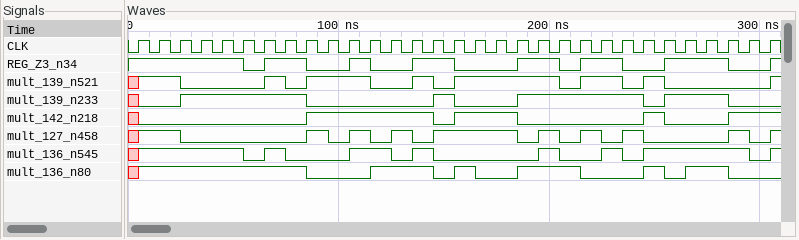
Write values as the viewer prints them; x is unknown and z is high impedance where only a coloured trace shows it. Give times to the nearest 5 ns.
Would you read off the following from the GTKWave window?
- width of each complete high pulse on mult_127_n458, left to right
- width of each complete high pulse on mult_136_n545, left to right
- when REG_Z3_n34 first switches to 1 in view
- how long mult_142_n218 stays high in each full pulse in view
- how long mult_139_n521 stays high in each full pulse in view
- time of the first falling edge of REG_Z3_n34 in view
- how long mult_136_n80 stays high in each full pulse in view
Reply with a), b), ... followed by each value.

a) 10 ns, 10 ns, 10 ns, 40 ns, 10 ns, 10 ns, 10 ns, 10 ns
b) 10 ns, 20 ns, 10 ns, 10 ns, 10 ns, 50 ns
c) 65 ns
d) 60 ns, 30 ns, 10 ns
e) 10 ns, 30 ns, 10 ns, 50 ns, 20 ns, 10 ns
f) 55 ns
g) 30 ns, 10 ns, 30 ns, 10 ns, 20 ns
